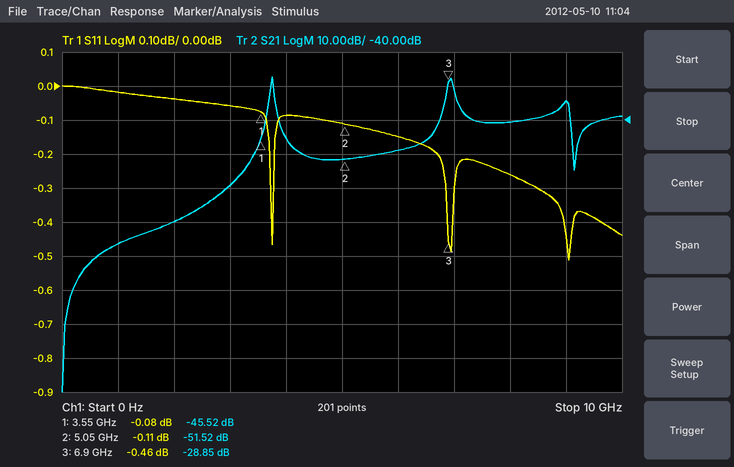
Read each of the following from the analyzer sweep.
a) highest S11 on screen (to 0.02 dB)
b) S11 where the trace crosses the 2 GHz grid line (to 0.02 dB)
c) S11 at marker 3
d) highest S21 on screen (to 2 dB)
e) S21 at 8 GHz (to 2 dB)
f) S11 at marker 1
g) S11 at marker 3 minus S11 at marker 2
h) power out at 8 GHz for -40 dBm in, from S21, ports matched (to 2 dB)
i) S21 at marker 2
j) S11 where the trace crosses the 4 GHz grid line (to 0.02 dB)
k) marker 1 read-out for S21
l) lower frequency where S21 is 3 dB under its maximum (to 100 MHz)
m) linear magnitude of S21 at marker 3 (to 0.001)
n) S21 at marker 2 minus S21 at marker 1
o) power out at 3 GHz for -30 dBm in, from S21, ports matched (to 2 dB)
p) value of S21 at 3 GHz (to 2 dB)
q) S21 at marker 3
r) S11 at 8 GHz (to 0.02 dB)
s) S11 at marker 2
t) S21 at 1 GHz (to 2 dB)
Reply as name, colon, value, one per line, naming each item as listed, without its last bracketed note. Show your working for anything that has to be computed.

highest S11 on screen: 0.00 dB
S11 where the trace crosses the 2 GHz grid line: -0.04 dB
S11 at marker 3: -0.46 dB
highest S21 on screen: -28 dB
S21 at 8 GHz: -40 dB
S11 at marker 1: -0.08 dB
S11 at marker 3 minus S11 at marker 2: -0.46 − (-0.11) = -0.35 dB
power out at 8 GHz for -40 dBm in, from S21, ports matched: -40 dBm + (-40 dB) = -80 dBm
S21 at marker 2: -51.52 dB
S11 where the trace crosses the 4 GHz grid line: -0.08 dB
marker 1 read-out for S21: -45.52 dB
lower frequency where S21 is 3 dB under its maximum: 3.7 GHz
linear magnitude of S21 at marker 3: 10^(-28.85/20) ≈ 0.036
S21 at marker 2 minus S21 at marker 1: -51.52 − (-45.52) = -6.00 dB
power out at 3 GHz for -30 dBm in, from S21, ports matched: -30 dBm + (-60 dB) = -90 dBm
value of S21 at 3 GHz: -60 dB
S21 at marker 3: -28.85 dB
S11 at 8 GHz: -0.26 dB
S11 at marker 2: -0.11 dB
S21 at 1 GHz: -76 dB
